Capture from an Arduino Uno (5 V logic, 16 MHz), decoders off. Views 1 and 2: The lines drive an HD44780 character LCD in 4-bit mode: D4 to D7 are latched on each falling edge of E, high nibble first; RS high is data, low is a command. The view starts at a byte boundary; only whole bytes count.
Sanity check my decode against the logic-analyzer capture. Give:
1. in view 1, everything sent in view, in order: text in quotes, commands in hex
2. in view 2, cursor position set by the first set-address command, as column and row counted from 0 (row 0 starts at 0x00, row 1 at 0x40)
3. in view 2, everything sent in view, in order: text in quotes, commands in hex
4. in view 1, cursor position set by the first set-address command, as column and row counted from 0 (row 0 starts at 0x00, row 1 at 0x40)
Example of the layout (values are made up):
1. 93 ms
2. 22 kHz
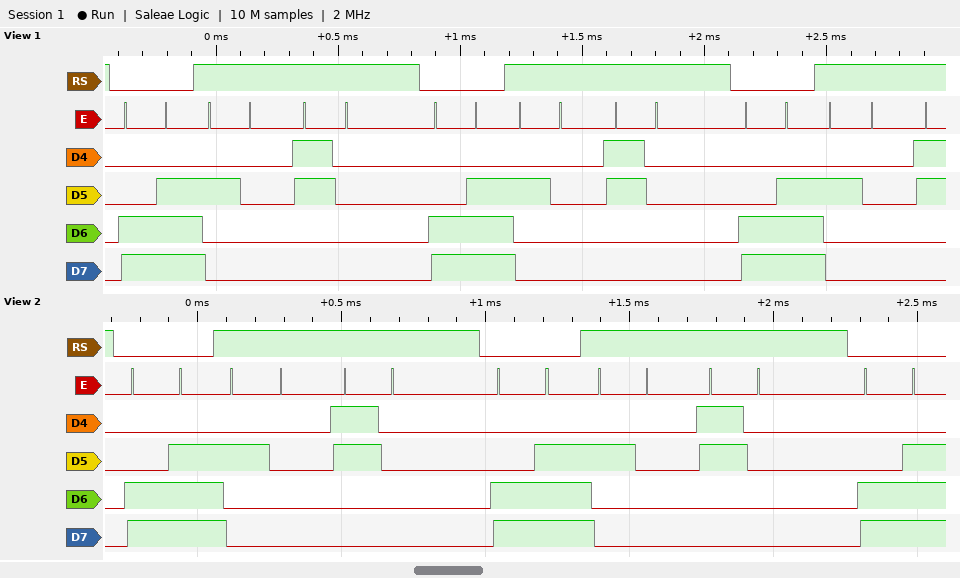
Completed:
1. 0xCE " 0" 0xCE " 0" 0xCE " "
2. column 14, row 1
3. 0xCE " 0" 0xCE " 0" 0xCE
4. column 14, row 1
